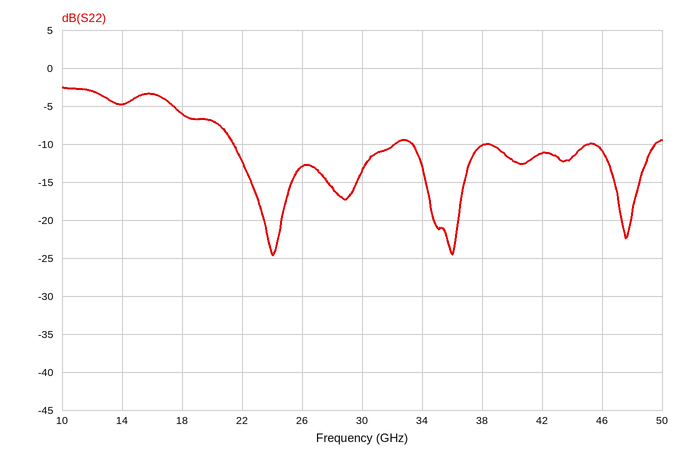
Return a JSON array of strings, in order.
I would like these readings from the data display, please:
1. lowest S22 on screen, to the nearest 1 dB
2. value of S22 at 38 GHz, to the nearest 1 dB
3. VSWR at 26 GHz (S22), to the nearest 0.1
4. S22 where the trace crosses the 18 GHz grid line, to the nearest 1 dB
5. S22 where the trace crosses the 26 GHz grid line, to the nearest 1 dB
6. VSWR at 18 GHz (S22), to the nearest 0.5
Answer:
["-25 dB", "-10 dB", "1.6", "-6 dB", "-13 dB", "3.0"]
